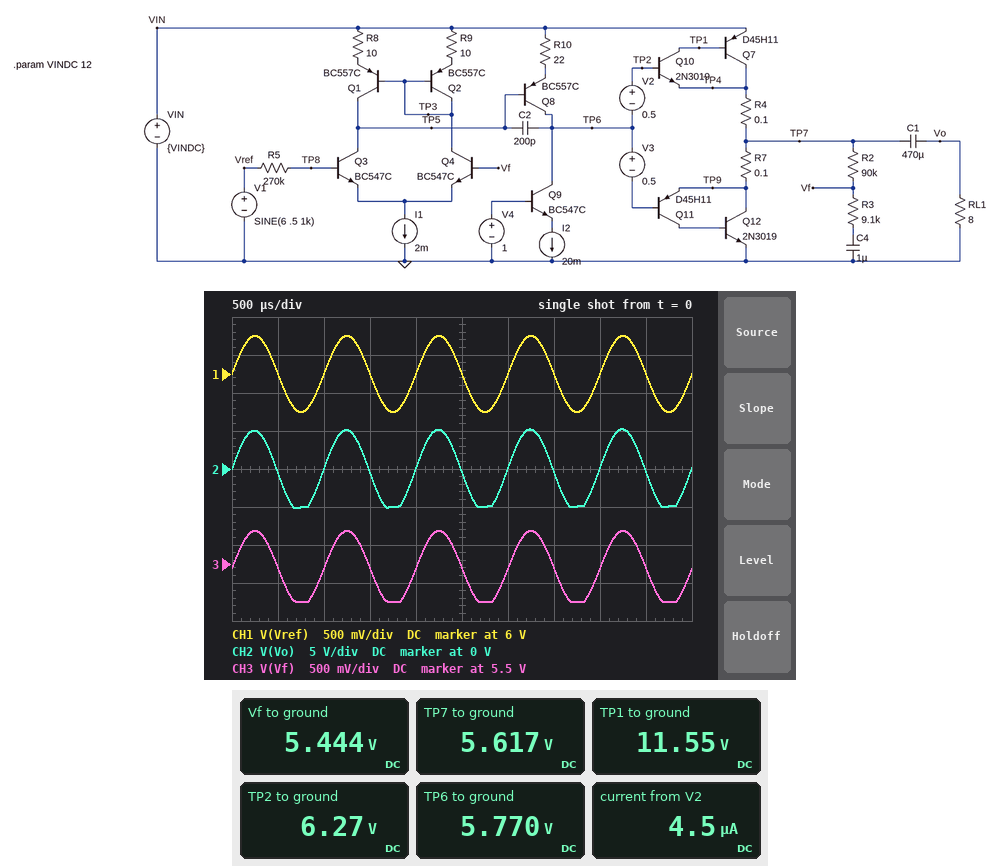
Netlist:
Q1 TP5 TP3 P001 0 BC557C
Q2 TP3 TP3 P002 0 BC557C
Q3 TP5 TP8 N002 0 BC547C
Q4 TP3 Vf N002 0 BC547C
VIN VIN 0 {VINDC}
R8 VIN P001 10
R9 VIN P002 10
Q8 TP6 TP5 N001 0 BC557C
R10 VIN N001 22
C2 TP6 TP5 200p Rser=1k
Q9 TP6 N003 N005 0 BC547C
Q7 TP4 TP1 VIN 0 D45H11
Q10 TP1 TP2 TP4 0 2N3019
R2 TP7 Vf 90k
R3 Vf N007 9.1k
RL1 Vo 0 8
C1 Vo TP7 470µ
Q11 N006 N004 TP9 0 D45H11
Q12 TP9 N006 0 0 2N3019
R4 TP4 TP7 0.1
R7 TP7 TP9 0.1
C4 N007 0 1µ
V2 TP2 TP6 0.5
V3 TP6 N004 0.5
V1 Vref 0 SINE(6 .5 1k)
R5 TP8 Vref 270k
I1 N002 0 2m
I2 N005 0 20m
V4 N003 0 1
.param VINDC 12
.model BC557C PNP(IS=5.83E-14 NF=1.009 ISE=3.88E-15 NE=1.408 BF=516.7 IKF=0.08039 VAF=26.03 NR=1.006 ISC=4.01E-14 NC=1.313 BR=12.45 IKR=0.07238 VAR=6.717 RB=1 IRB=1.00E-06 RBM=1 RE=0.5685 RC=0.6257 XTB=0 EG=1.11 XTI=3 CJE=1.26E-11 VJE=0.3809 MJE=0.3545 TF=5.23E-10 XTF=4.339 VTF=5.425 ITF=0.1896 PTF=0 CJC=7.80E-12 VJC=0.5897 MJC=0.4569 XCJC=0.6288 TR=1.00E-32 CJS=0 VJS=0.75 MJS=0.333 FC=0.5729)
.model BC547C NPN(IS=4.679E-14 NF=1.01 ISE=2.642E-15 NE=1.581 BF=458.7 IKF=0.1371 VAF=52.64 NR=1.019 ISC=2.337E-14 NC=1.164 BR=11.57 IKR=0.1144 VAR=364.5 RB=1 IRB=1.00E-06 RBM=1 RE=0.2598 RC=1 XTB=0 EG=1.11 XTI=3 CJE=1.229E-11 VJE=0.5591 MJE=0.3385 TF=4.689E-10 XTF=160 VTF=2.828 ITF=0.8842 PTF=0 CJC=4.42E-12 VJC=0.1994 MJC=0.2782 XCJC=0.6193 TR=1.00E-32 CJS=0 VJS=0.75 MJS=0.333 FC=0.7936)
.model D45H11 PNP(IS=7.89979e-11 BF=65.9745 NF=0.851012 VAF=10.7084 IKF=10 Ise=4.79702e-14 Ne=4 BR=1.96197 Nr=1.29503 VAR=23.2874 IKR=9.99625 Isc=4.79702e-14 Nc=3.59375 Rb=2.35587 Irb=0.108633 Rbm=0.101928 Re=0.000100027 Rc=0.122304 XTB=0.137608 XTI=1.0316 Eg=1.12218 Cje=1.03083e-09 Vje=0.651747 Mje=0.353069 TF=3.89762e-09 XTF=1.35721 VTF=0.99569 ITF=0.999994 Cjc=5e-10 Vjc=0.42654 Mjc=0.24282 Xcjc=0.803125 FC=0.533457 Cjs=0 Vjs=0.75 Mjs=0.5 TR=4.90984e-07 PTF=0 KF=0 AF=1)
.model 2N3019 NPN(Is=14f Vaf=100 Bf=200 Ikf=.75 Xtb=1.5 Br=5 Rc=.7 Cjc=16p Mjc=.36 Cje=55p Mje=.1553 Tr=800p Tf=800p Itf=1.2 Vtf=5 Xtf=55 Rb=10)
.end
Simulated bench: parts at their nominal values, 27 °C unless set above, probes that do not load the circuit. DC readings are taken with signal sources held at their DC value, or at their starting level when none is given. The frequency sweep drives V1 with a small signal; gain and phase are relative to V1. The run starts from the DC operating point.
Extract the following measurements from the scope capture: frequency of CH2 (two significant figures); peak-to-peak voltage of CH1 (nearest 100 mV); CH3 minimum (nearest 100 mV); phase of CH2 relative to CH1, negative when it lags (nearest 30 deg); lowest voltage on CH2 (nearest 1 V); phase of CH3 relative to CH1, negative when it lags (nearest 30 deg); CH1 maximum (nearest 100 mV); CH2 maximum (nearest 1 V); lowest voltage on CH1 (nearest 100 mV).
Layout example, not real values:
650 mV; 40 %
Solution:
1.0 kHz; 1.0 V; 5.0 V; 0 deg; -5 V; 0 deg; 6.5 V; 5 V; 5.5 V
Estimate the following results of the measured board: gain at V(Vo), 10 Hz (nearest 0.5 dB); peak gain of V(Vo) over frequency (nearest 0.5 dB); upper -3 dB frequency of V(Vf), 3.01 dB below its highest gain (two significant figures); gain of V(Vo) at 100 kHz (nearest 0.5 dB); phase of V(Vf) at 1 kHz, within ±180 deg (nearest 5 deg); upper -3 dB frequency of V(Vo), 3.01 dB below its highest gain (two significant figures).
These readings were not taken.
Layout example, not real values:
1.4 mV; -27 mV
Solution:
2.0 dB; 20.5 dB; 170 kHz; 19.5 dB; 0 deg; 170 kHz
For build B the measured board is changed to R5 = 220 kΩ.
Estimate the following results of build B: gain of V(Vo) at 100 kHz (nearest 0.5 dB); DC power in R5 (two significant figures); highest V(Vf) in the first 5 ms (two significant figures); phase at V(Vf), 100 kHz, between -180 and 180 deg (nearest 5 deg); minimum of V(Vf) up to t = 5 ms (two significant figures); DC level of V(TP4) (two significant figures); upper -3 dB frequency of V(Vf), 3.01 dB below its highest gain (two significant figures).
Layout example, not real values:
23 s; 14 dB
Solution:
20.0 dB; 930 nW; 6.0 V; -35 deg; 5.1 V; 5.7 V; 200 kHz
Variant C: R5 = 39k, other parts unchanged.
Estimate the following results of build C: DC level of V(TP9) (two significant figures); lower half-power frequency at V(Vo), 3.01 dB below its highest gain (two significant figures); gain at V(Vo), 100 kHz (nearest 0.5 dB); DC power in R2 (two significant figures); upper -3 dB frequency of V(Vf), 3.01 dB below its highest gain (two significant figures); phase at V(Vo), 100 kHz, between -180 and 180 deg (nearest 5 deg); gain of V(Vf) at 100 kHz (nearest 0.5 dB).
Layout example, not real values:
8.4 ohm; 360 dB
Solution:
6.1 V; 55 Hz; 21.0 dB; 340 nW; 670 kHz; -10 deg; 0 dB
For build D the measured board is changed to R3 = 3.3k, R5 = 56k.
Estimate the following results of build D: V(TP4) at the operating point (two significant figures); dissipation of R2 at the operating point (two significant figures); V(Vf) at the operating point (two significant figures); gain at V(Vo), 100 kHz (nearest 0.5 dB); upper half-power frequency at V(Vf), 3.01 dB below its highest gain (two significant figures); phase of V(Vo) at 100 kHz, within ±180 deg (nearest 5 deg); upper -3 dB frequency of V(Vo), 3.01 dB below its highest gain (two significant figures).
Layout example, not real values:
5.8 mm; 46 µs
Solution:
6.1 V; 340 nW; 5.9 V; 29.0 dB; 310 kHz; -25 deg; 320 kHz
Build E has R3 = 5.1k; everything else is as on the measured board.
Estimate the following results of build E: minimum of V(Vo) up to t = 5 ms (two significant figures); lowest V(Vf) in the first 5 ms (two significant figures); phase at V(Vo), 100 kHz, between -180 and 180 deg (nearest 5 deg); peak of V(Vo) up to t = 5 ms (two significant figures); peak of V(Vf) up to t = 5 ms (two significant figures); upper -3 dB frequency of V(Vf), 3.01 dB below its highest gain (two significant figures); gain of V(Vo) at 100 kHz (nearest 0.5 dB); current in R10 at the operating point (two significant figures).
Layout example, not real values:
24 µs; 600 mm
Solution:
-5.3 V; 5.2 V; -55 deg; 5.6 V; 5.8 V; 120 kHz; 23.0 dB; 20 mA
